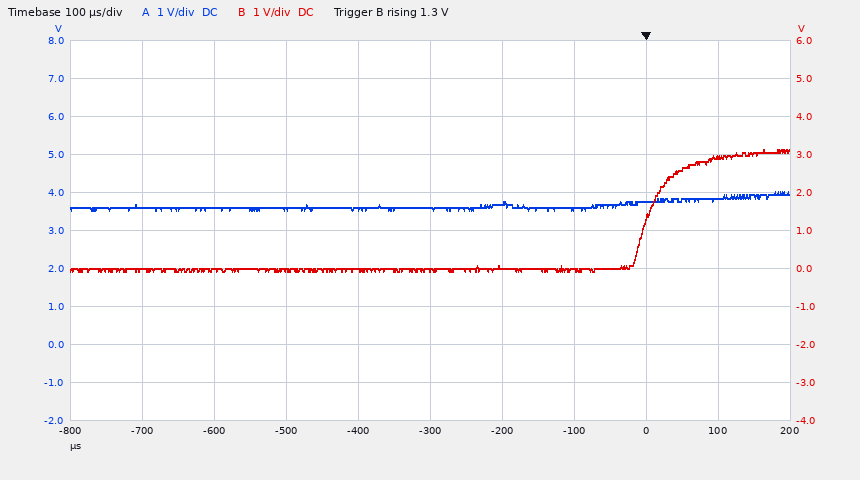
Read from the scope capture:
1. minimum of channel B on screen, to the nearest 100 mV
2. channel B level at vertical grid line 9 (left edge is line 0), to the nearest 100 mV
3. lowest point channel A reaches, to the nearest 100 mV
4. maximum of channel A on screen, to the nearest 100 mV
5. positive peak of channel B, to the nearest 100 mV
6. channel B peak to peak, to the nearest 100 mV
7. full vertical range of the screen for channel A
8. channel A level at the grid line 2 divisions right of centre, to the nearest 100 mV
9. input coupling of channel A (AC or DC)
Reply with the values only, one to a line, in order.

-100 mV
2.9 V
3.5 V
4.0 V
3.1 V
3.2 V
10 V
3.6 V
DC
